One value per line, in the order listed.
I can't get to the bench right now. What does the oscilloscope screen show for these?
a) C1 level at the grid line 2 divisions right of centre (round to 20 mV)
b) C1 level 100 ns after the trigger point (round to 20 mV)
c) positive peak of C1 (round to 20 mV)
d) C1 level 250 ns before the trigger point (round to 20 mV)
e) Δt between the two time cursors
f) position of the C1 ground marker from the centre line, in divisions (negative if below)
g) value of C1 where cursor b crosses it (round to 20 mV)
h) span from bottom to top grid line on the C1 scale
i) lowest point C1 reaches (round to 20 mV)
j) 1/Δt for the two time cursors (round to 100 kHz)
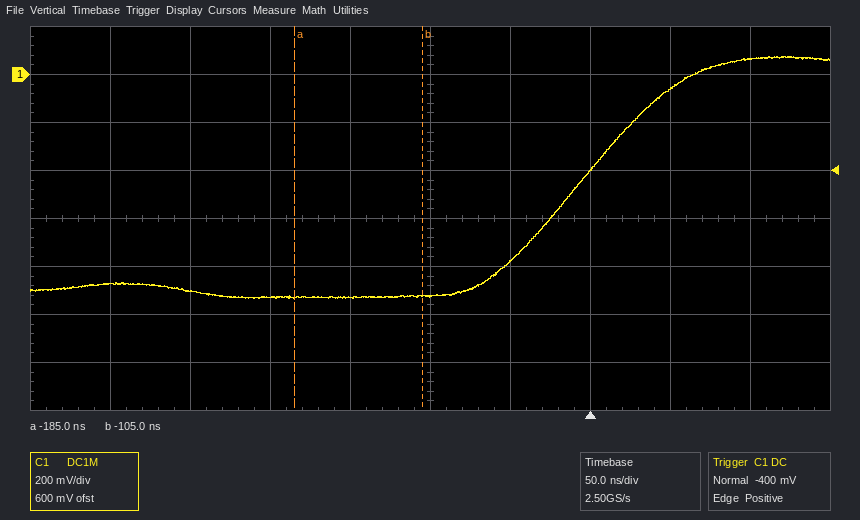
-400 mV
60 mV
80 mV
-900 mV
80 ns
+3.0 div
-920 mV
1.6 V
-940 mV
12.5 MHz
